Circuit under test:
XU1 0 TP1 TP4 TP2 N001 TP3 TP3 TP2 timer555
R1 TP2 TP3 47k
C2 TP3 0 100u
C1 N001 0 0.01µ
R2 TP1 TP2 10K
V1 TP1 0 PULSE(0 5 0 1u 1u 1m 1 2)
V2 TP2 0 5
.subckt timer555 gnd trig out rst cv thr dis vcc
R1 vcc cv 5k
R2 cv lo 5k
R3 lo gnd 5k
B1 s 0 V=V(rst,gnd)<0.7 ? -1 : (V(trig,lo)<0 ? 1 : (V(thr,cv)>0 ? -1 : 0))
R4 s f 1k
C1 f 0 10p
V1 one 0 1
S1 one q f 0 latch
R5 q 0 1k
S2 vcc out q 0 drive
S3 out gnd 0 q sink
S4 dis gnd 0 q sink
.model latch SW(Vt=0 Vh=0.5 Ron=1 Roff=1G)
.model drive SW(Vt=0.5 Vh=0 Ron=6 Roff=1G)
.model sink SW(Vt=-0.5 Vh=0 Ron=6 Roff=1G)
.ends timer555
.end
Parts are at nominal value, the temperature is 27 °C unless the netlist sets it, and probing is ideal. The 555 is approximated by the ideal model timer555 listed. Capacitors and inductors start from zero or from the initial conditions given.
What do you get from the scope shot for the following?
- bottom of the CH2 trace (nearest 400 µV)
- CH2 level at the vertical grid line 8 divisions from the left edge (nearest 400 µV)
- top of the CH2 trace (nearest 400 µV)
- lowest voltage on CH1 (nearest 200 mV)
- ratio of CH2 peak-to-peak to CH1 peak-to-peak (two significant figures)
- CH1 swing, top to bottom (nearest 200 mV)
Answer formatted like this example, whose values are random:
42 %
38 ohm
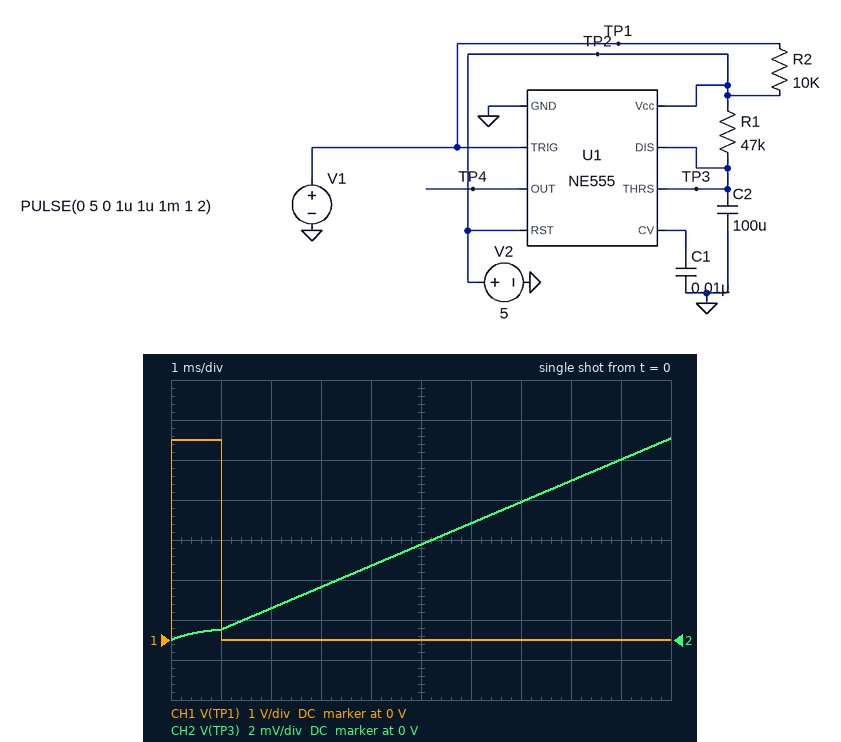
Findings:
0 V
8.0 mV
10.0 mV
0 V
0.0020
5.0 V
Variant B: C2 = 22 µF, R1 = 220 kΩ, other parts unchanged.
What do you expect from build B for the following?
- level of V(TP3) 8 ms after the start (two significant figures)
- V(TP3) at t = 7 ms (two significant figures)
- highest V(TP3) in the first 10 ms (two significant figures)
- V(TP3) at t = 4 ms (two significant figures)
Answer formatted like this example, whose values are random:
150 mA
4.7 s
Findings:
7.4 mV
6.3 mV
9.4 mV
3.2 mV
